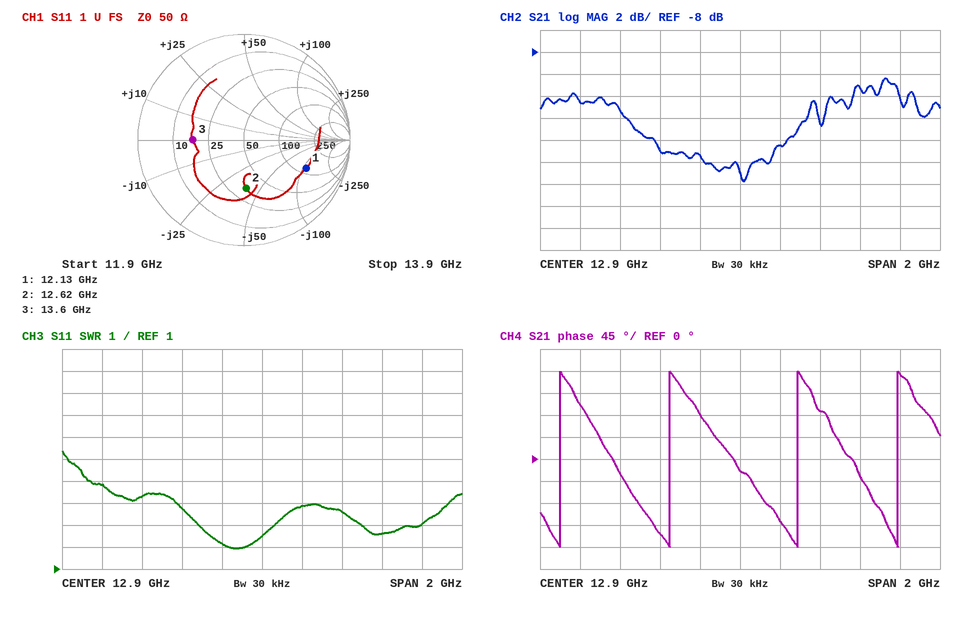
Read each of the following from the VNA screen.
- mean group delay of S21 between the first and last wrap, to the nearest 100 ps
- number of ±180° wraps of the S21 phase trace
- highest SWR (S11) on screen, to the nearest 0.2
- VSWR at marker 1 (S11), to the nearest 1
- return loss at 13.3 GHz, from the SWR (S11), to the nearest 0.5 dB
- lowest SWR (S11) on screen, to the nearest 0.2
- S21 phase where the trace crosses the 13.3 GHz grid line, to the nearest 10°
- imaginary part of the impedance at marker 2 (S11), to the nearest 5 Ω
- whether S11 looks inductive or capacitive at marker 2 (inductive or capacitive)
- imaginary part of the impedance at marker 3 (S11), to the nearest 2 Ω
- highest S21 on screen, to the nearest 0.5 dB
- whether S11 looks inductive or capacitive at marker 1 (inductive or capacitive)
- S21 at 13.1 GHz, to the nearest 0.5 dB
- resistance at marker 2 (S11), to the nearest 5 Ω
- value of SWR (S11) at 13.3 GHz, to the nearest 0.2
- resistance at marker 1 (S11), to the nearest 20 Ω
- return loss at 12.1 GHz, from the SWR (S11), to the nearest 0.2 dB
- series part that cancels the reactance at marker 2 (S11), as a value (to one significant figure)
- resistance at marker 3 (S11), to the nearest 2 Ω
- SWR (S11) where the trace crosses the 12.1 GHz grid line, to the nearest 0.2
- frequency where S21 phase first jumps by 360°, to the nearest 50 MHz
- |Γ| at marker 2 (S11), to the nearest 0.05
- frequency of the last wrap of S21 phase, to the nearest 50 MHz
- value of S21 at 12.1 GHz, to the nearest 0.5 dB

1.8 ns
4
6.4
5
5.0 dB
2.0
100°
-40 Ω
capacitive
0 Ω
-10.5 dB
capacitive
-16.5 dB
35 Ω
3.6
120 Ω
3.6 dB
500 pH
18 Ω
4.8
12.00 GHz
0.45
13.70 GHz
-12.5 dB
